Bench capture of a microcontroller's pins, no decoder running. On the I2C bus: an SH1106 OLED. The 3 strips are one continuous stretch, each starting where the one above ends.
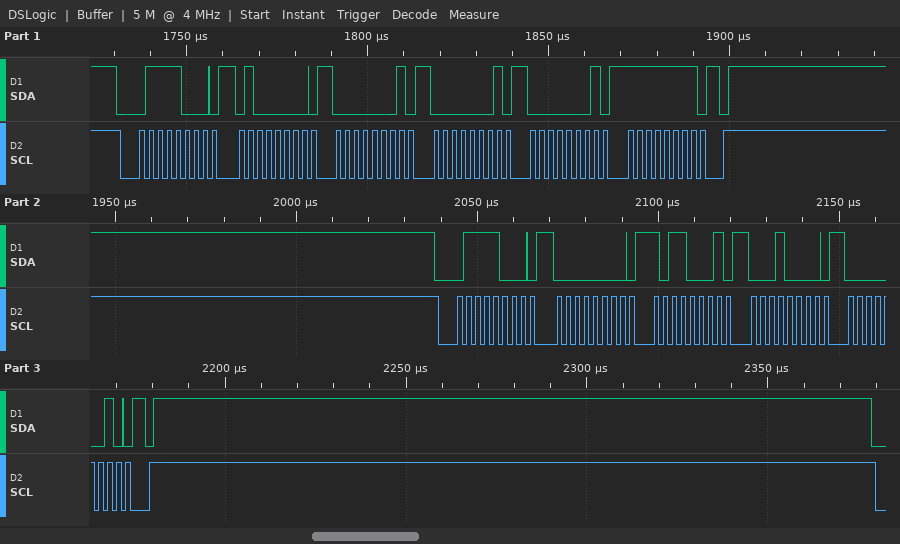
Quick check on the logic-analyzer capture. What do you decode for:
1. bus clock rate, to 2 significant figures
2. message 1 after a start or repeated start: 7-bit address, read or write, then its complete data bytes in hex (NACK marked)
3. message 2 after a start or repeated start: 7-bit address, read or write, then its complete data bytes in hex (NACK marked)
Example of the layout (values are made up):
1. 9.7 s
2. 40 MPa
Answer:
1. 400 kHz
2. 0x3C write: 40 01 01 01 FF
3. 0x3C write: 00 B1 10 02
